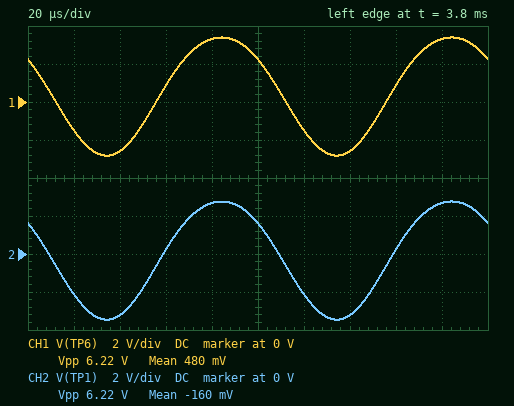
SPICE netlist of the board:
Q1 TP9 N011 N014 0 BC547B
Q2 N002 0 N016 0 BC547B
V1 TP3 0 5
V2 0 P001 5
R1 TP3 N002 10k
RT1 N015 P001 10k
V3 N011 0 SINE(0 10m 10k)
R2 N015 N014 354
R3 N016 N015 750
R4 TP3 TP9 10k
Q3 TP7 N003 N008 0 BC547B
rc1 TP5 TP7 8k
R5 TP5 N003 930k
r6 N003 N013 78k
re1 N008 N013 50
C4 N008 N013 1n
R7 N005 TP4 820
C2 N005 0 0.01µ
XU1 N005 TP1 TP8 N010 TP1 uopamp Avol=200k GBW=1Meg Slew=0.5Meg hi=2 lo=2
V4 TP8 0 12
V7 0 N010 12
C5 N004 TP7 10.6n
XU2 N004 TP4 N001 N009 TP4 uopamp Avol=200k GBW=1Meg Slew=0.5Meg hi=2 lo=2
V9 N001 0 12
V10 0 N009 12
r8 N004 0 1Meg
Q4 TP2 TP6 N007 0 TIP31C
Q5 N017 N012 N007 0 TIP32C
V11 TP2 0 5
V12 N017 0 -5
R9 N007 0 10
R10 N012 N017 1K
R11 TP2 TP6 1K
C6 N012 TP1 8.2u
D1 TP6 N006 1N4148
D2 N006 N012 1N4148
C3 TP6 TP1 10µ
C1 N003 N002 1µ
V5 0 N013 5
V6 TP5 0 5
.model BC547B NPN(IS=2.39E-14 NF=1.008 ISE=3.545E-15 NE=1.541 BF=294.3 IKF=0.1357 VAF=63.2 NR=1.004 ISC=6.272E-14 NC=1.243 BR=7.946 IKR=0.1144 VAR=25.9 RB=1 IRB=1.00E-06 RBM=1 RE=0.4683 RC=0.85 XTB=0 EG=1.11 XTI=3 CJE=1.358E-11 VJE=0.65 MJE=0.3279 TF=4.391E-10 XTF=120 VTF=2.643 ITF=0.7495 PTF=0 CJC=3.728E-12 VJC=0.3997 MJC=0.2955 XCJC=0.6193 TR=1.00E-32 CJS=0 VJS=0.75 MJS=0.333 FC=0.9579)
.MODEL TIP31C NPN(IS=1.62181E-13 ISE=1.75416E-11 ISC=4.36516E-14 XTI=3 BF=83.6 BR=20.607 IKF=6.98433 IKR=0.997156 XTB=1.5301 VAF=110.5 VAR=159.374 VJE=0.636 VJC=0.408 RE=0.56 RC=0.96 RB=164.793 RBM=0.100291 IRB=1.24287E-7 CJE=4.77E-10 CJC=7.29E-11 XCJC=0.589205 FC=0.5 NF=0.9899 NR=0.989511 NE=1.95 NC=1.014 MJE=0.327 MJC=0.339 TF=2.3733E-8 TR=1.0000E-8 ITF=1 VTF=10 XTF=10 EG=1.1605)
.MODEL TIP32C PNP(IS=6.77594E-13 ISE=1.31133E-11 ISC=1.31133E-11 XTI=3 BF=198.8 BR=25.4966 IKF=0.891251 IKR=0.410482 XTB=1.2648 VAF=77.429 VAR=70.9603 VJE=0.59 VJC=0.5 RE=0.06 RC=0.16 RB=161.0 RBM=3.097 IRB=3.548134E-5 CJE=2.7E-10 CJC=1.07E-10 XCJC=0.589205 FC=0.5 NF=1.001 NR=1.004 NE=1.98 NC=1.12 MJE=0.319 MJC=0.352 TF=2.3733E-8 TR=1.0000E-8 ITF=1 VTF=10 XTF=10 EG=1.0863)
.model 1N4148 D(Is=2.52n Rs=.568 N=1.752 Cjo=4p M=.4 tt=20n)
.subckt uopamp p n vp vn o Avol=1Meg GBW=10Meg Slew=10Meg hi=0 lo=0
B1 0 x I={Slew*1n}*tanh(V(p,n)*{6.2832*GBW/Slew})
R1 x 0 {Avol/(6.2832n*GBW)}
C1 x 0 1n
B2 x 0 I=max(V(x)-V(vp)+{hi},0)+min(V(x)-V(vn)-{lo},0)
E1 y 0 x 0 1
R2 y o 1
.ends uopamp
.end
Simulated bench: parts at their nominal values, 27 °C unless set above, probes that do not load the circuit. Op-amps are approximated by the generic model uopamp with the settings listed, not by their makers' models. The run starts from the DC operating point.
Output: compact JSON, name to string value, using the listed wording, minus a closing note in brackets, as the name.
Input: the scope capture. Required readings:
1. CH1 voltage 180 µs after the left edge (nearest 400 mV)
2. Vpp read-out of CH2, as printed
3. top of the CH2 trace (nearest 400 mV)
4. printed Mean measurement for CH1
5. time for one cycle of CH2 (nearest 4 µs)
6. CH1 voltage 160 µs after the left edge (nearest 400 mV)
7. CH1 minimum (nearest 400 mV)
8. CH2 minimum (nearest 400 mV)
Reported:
{"CH1 voltage 180 µs after the left edge": "3.2 V", "Vpp read-out of CH2, as printed": "6.22 V", "top of the CH2 trace": "2.8 V", "printed Mean measurement for CH1": "480 mV", "time for one cycle of CH2": "100 µs", "CH1 voltage 160 µs after the left edge": "800 mV", "CH1 minimum": "-2.8 V", "CH2 minimum": "-3.6 V"}
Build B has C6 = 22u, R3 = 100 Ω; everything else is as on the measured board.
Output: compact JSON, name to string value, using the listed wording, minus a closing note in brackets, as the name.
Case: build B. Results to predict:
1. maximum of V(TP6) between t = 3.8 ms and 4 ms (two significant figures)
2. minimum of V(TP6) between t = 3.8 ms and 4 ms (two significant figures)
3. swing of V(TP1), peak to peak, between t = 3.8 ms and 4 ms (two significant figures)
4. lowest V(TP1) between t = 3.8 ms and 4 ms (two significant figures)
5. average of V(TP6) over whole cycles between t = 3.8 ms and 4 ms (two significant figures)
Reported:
{"maximum of V(TP6) between t = 3.8 ms and 4 ms": "4.8 V", "minimum of V(TP6) between t = 3.8 ms and 4 ms": "-4.3 V", "swing of V(TP1), peak to peak, between t = 3.8 ms and 4 ms": "9.1 V", "lowest V(TP1) between t = 3.8 ms and 4 ms": "-5.2 V", "average of V(TP6) over whole cycles between t = 3.8 ms and 4 ms": "480 mV"}
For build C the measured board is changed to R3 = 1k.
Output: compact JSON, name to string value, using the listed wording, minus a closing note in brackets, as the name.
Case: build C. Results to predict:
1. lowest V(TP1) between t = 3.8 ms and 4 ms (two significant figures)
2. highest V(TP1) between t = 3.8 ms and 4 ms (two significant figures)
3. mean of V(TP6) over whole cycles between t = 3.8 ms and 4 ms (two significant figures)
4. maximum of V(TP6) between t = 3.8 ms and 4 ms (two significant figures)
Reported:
{"lowest V(TP1) between t = 3.8 ms and 4 ms": "-2.9 V", "highest V(TP1) between t = 3.8 ms and 4 ms": "2.4 V", "mean of V(TP6) over whole cycles between t = 3.8 ms and 4 ms": "510 mV", "maximum of V(TP6) between t = 3.8 ms and 4 ms": "3.0 V"}
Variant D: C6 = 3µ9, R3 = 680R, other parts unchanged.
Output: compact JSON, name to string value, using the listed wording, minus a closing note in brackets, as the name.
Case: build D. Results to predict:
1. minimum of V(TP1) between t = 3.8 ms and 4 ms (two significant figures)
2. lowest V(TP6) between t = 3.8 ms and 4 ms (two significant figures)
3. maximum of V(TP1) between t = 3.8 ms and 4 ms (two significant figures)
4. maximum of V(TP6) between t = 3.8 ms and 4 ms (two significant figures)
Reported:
{"minimum of V(TP1) between t = 3.8 ms and 4 ms": "-3.7 V", "lowest V(TP6) between t = 3.8 ms and 4 ms": "-3.0 V", "maximum of V(TP1) between t = 3.8 ms and 4 ms": "2.9 V", "maximum of V(TP6) between t = 3.8 ms and 4 ms": "3.5 V"}
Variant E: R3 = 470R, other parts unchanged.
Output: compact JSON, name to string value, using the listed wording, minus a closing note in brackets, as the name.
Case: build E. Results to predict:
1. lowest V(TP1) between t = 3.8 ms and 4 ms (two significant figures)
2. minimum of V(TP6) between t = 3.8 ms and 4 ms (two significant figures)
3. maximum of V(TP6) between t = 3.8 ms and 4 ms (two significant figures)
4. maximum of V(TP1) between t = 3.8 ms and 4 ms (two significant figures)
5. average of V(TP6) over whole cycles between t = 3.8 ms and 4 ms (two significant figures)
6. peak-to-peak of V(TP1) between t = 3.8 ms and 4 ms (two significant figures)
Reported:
{"lowest V(TP1) between t = 3.8 ms and 4 ms": "-4.5 V", "minimum of V(TP6) between t = 3.8 ms and 4 ms": "-3.8 V", "maximum of V(TP6) between t = 3.8 ms and 4 ms": "4.0 V", "maximum of V(TP1) between t = 3.8 ms and 4 ms": "3.3 V", "average of V(TP6) over whole cycles between t = 3.8 ms and 4 ms": "410 mV", "peak-to-peak of V(TP1) between t = 3.8 ms and 4 ms": "7.8 V"}
